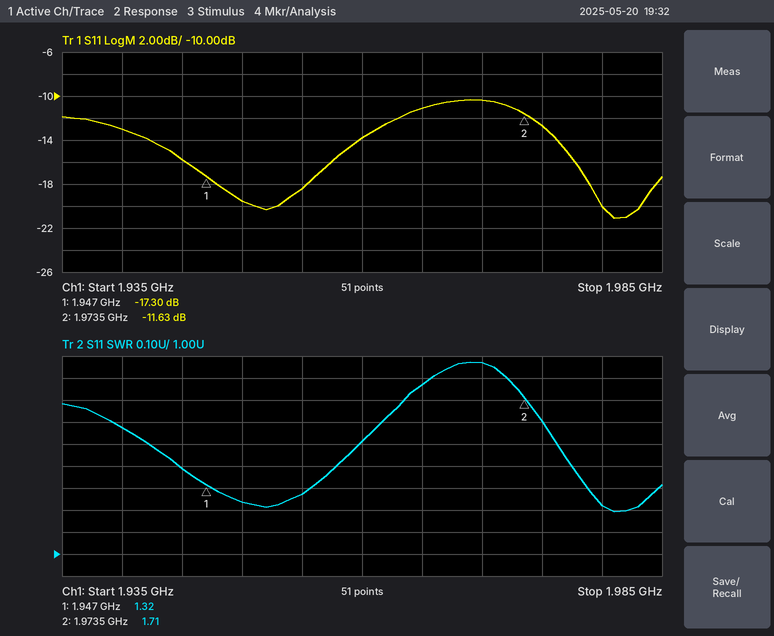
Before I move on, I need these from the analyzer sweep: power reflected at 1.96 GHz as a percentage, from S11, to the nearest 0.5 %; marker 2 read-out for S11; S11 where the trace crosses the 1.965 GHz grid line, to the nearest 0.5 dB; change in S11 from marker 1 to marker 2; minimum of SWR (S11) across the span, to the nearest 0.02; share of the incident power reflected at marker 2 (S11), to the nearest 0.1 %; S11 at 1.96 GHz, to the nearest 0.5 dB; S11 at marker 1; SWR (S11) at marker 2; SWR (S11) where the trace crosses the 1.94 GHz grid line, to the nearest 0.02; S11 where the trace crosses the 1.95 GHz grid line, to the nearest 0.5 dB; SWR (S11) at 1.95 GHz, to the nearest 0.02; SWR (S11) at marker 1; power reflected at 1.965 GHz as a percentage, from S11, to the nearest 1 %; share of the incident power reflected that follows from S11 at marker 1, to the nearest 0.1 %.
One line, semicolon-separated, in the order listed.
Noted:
4.0 %; -11.63 dB; -11.0 dB; 5.67 dB; 1.20; 6.9 %; -14.0 dB; -17.30 dB; 1.71; 1.58; -19.5 dB; 1.24; 1.32; 8 %; 1.9 %
